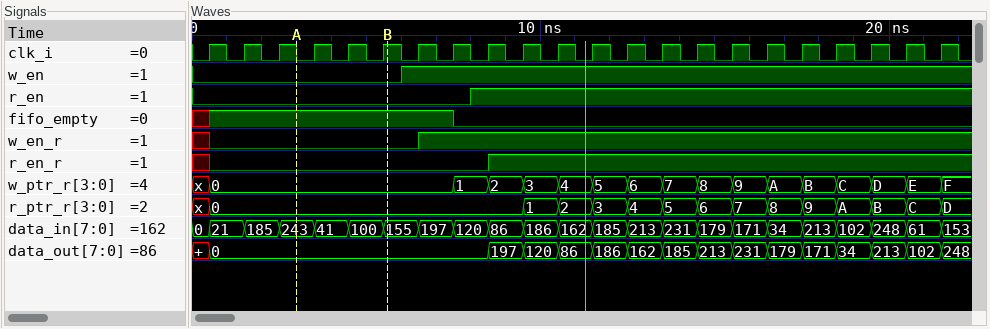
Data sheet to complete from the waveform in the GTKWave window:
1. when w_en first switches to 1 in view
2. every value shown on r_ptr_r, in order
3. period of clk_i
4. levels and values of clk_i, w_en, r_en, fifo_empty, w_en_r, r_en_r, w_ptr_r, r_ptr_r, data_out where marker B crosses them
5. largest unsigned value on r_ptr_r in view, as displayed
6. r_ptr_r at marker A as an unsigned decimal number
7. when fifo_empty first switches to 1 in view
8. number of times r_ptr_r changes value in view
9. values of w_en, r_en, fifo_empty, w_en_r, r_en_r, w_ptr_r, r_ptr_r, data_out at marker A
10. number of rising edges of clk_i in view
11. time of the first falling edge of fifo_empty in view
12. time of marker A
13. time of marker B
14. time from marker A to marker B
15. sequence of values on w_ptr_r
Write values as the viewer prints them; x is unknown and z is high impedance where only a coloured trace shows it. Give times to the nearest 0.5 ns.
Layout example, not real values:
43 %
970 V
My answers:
6 ns
x, 0, 1, 2, 3, 4, 5, 6, 7, 8, 9, A, B, C, D
1 ns
clk_i=1, w_en=0, r_en=0, fifo_empty=1, w_en_r=0, r_en_r=0, w_ptr_r=0, r_ptr_r=0, data_out=0
D
0
0.5 ns
14
w_en=0, r_en=0, fifo_empty=1, w_en_r=0, r_en_r=0, w_ptr_r=0, r_ptr_r=0, data_out=0
22
7.5 ns
3 ns
5.5 ns
2.5 ns
x, 0, 1, 2, 3, 4, 5, 6, 7, 8, 9, A, B, C, D, E, F
